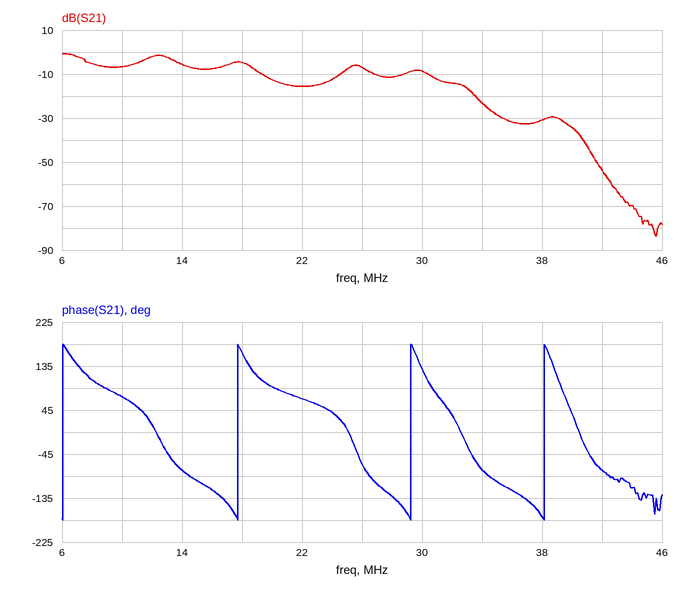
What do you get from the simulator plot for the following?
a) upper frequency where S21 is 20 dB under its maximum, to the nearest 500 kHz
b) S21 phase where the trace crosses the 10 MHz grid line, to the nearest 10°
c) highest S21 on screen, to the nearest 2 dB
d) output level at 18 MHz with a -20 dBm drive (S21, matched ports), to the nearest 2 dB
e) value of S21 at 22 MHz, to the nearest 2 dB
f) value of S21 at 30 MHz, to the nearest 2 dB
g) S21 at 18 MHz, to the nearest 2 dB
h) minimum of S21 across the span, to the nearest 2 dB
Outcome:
33.5 MHz
70°
0 dB
-24 dBm
-16 dB
-8 dB
-4 dB
-84 dB
